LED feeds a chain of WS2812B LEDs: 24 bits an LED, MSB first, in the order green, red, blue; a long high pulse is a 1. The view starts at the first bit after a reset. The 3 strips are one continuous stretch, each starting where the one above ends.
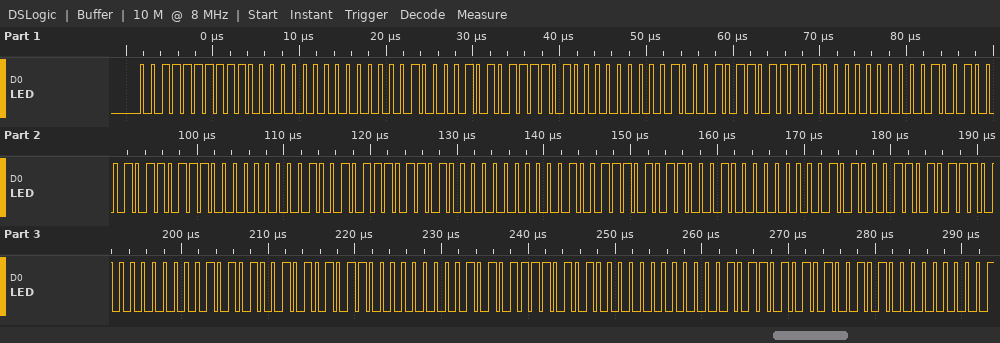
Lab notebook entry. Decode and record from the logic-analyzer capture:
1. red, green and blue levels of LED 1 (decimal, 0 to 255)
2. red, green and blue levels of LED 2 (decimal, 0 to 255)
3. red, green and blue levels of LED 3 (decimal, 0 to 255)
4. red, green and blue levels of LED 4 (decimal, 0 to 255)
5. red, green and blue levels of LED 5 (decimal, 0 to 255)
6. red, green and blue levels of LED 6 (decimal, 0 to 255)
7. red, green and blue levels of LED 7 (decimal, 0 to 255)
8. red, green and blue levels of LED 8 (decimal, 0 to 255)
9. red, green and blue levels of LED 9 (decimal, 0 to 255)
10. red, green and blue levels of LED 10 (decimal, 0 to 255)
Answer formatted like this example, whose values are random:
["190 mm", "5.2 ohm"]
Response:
["192, 63, 0", "189, 66, 0", "186, 69, 0", "183, 72, 0", "180, 75, 0", "177, 78, 0", "174, 81, 0", "171, 84, 0", "168, 87, 0", "165, 90, 0"]
